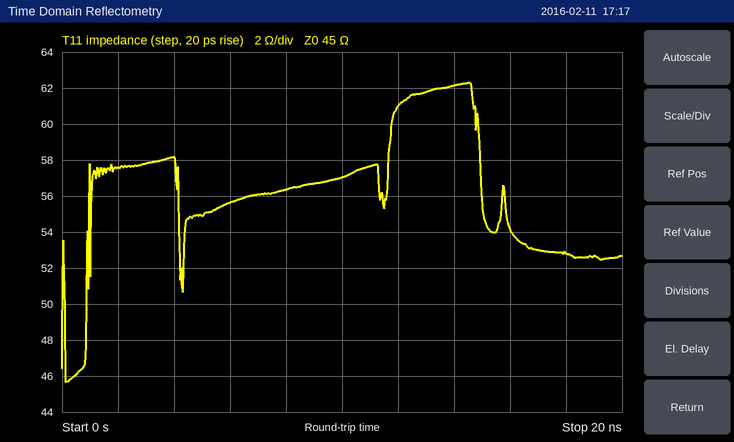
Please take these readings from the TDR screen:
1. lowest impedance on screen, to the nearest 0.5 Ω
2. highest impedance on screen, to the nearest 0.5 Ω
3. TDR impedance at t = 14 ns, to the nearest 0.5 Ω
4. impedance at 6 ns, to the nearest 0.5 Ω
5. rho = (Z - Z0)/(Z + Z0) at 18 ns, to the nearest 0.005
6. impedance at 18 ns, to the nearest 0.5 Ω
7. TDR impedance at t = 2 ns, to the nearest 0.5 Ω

45.5 Ω
62.5 Ω
62.0 Ω
55.5 Ω
+0.080
53.0 Ω
57.5 Ω
